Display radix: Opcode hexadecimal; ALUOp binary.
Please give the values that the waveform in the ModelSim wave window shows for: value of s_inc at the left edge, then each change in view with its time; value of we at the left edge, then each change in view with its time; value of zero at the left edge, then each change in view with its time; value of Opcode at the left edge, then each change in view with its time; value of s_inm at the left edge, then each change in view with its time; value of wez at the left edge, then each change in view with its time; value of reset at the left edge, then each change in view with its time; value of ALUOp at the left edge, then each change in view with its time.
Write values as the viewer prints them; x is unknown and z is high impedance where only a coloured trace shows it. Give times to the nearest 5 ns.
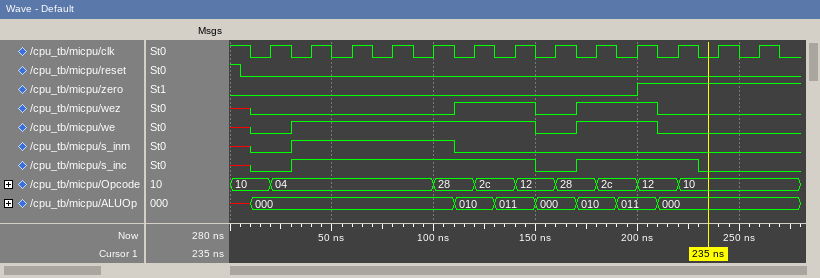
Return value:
x, 0 at 10 ns, 1 at 30 ns, 0 at 150 ns, 1 at 170 ns, 0 at 230 ns
x, 0 at 10 ns, 1 at 30 ns, 0 at 150 ns, 1 at 170 ns, 0 at 210 ns
0, 1 at 200 ns
10, 04 at 20 ns, 28 at 100 ns, 2c at 120 ns, 12 at 140 ns, 28 at 160 ns, 2c at 180 ns, 12 at 200 ns, 10 at 220 ns
x, 0 at 10 ns, 1 at 30 ns, 0 at 110 ns
x, 0 at 10 ns, 1 at 110 ns, 0 at 150 ns, 1 at 170 ns, 0 at 210 ns
1, 0 at 5 ns
x, 000 at 10 ns, 010 at 110 ns, 011 at 130 ns, 000 at 150 ns, 010 at 170 ns, 011 at 190 ns, 000 at 210 ns
